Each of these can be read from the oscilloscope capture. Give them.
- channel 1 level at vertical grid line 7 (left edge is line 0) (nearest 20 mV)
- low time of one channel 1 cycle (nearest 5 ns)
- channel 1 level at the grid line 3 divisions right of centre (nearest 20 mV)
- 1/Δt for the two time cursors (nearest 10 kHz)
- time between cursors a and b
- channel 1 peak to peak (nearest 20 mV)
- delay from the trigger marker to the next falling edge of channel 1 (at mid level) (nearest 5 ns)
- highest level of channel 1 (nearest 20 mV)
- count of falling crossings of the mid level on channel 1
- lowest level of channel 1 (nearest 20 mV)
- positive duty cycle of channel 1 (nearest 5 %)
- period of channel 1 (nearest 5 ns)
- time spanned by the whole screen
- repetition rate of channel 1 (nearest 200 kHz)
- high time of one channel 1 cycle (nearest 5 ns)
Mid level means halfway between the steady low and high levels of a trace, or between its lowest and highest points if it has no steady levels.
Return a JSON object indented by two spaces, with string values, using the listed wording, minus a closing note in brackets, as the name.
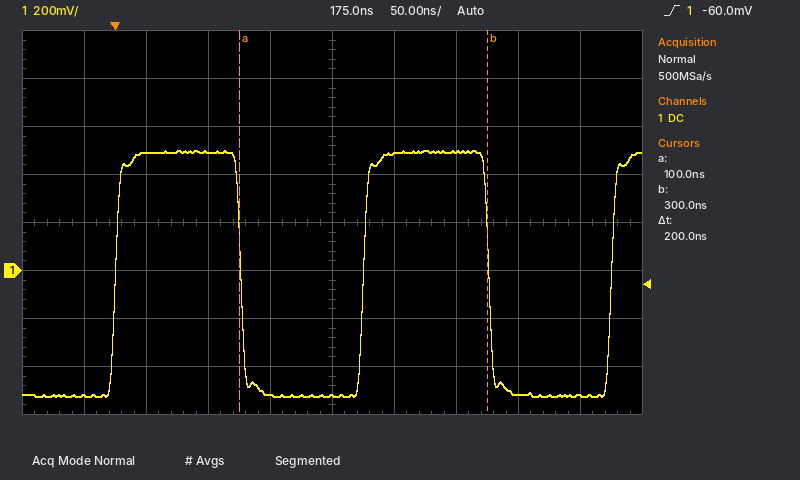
{
  "channel 1 level at vertical grid line 7 (left edge is line 0)": "500 mV",
  "low time of one channel 1 cycle": "100 ns",
  "channel 1 level at the grid line 3 divisions right of centre": "-520 mV",
  "1/Δt for the two time cursors": "5.00 MHz",
  "time between cursors a and b": "200 ns",
  "channel 1 peak to peak": "1.02 V",
  "delay from the trigger marker to the next falling edge of channel 1 (at mid level)": "100 ns",
  "highest level of channel 1": "500 mV",
  "count of falling crossings of the mid level on channel 1": "2",
  "lowest level of channel 1": "-520 mV",
  "positive duty cycle of channel 1": "50 %",
  "period of channel 1": "200 ns",
  "time spanned by the whole screen": "500 ns",
  "repetition rate of channel 1": "5.0 MHz",
  "high time of one channel 1 cycle": "100 ns"
}
